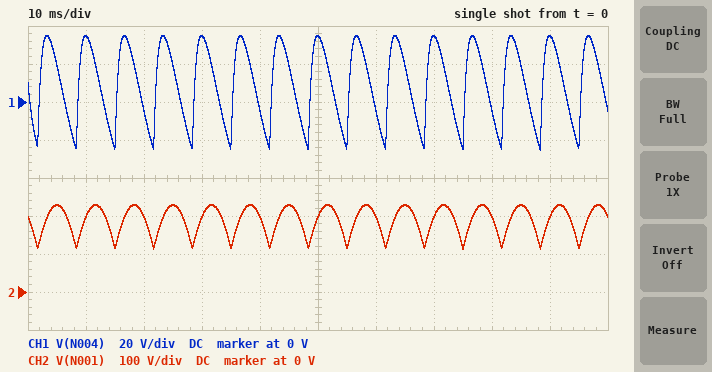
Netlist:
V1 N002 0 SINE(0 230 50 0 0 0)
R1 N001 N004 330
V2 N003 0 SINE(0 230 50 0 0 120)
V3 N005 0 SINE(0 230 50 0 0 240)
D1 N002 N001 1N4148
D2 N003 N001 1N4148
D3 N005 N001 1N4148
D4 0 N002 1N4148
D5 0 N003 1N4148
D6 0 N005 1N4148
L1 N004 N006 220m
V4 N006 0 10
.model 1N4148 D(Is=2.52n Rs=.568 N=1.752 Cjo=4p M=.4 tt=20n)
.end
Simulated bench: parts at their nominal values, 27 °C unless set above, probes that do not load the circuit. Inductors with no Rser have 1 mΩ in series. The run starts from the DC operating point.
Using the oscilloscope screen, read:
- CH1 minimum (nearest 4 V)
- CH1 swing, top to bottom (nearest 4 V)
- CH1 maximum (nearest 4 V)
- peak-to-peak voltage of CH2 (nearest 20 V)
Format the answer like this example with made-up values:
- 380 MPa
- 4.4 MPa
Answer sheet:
- -24 V
- 60 V
- 36 V
- 120 V
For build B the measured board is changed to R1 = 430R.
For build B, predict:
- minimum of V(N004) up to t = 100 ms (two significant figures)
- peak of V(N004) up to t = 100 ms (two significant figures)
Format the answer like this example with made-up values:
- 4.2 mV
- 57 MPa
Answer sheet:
- -18 V
- 31 V
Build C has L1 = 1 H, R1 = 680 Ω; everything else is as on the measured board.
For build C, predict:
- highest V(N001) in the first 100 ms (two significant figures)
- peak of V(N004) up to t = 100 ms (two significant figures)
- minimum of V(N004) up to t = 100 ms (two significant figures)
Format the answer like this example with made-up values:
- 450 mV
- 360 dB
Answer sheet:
- 230 V
- 45 V
- -47 V
